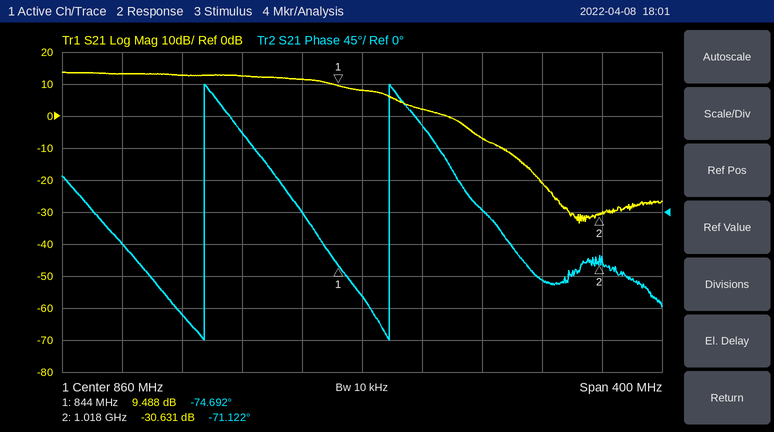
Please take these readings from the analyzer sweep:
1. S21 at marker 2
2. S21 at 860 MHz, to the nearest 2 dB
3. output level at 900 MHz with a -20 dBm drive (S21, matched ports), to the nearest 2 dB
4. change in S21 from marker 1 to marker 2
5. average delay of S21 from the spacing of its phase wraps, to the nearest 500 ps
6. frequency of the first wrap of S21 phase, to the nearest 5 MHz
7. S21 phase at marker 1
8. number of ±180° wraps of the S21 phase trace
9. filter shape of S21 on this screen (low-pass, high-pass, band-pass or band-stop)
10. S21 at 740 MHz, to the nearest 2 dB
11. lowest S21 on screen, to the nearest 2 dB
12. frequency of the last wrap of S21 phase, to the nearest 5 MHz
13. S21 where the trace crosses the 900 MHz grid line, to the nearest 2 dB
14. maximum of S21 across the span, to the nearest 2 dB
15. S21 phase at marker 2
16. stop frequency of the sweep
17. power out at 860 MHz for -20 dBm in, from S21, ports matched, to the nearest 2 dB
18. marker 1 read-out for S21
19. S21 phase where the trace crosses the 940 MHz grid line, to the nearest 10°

-30.631 dB
8 dB
-18 dBm
-40.119 dB
8.0 ns
755 MHz
-74.692°
2
low-pass
12 dB
-34 dB
880 MHz
2 dB
14 dB
-71.122°
1.06 GHz
-12 dBm
9.488 dB
0°
